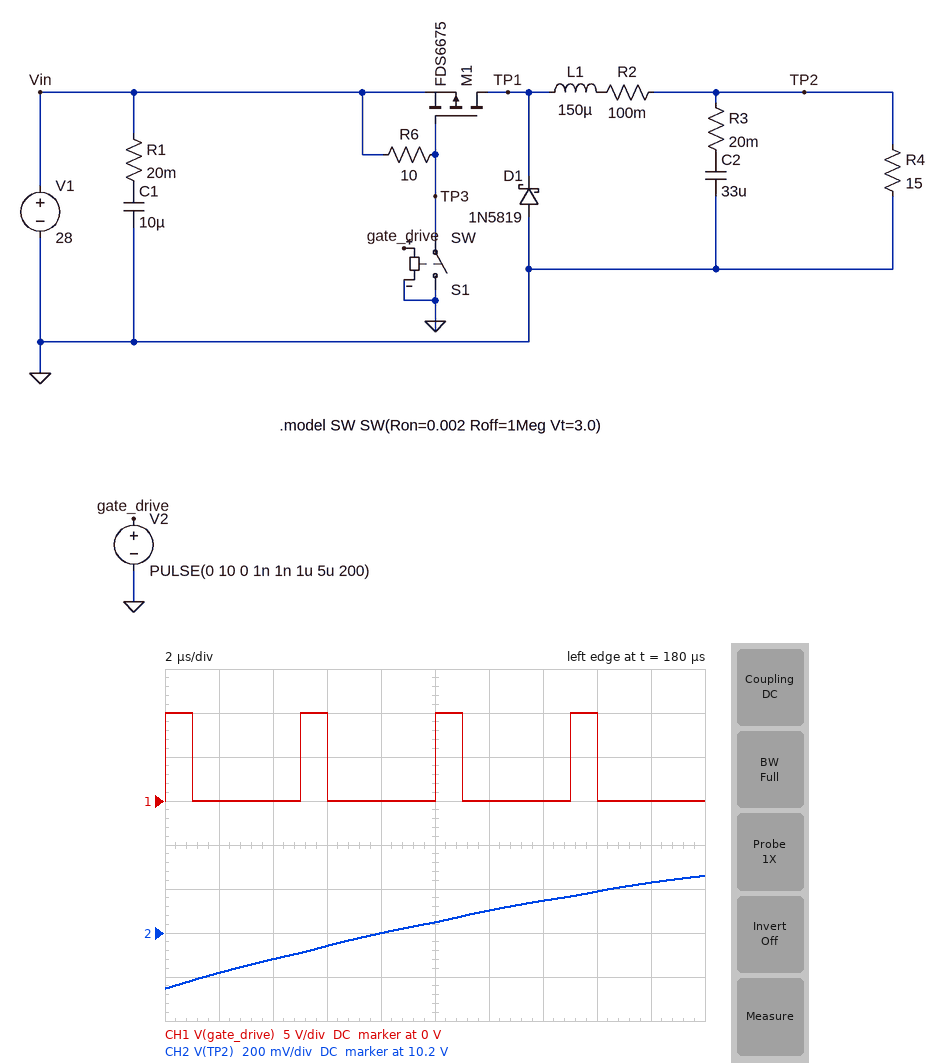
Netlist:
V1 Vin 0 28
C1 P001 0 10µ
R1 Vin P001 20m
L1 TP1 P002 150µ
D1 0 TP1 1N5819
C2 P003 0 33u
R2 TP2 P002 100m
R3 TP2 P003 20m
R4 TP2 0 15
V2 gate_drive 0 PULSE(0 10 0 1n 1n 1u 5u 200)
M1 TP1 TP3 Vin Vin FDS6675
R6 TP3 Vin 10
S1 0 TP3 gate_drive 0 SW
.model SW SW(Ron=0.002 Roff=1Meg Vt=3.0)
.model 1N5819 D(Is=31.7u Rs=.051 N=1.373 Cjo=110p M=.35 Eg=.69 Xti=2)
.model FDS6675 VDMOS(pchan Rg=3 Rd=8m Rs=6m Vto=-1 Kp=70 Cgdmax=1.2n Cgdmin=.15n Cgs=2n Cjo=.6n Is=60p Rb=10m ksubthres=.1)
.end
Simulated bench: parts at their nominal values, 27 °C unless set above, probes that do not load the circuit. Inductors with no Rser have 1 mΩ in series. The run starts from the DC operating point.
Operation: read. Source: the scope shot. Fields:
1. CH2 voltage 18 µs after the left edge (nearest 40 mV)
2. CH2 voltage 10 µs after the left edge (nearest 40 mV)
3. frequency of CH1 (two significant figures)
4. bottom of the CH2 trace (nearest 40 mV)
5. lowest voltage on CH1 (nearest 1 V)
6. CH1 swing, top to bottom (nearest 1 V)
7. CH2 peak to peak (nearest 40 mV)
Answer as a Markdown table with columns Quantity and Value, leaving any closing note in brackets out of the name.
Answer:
| Quantity | Value |
|---|---|
| CH2 voltage 18 µs after the left edge | 10.44 V |
| CH2 voltage 10 µs after the left edge | 10.24 V |
| frequency of CH1 | 200 kHz |
| bottom of the CH2 trace | 9.96 V |
| lowest voltage on CH1 | 0 V |
| CH1 swing, top to bottom | 10 V |
| CH2 peak to peak | 520 mV |
